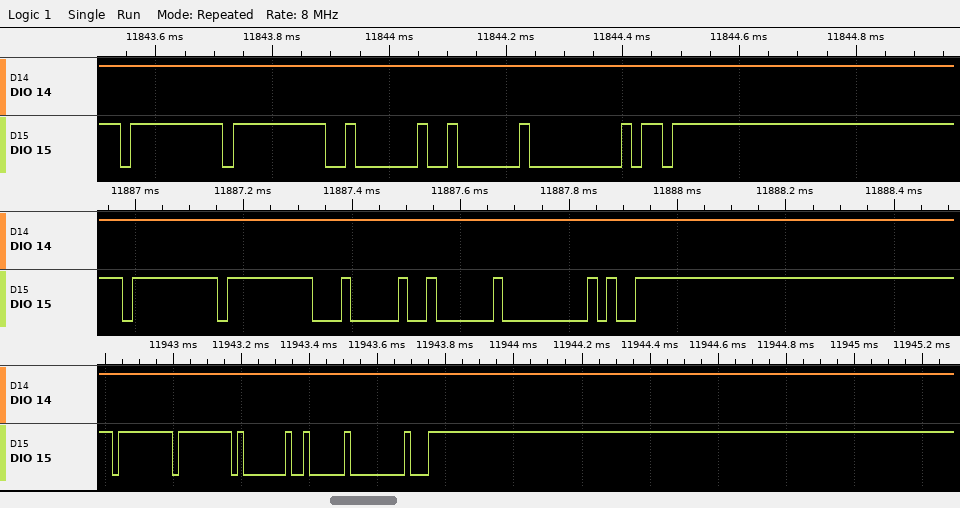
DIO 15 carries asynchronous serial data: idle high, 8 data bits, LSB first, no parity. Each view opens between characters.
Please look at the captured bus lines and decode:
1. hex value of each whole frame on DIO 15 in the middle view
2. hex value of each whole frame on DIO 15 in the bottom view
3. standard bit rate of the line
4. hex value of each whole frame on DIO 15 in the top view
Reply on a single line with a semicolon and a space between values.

FF, FF, 04, 02, 00, F9; FF, FF, 01, 02, 00, FC; 57600 baud; FF, FF, 02, 02, 00, FB
